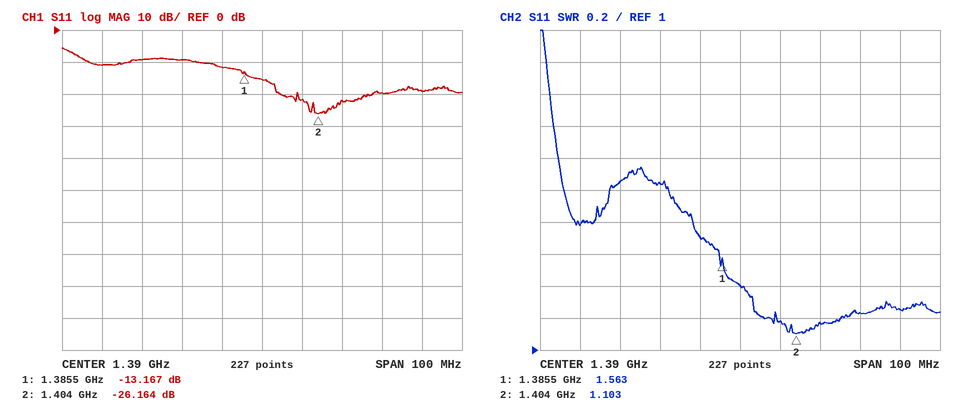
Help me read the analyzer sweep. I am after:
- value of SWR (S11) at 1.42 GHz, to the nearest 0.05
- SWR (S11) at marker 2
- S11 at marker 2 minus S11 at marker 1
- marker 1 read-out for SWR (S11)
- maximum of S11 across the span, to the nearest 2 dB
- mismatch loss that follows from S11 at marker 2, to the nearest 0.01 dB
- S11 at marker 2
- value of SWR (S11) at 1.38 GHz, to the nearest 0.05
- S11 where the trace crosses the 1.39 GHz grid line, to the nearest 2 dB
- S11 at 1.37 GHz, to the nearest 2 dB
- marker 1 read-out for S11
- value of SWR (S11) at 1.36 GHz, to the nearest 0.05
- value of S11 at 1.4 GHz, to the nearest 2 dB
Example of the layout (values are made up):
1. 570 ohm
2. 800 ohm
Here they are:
1. 1.25
2. 1.103
3. -12.997 dB
4. 1.563
5. -6 dB
6. 0.01 dB
7. -26.164 dB
8. 1.70
9. -16 dB
10. -10 dB
11. -13.167 dB
12. 2.05
13. -22 dB
